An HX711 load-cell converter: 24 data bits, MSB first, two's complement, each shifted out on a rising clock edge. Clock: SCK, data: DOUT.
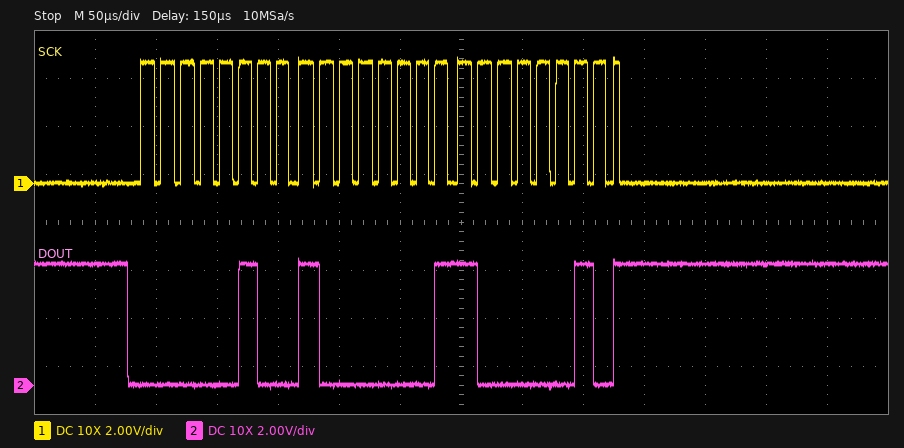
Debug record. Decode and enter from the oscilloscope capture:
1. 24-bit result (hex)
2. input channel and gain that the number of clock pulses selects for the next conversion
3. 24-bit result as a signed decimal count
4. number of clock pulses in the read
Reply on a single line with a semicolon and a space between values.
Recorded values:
0x048182; channel A, gain 128; 295298; 25
